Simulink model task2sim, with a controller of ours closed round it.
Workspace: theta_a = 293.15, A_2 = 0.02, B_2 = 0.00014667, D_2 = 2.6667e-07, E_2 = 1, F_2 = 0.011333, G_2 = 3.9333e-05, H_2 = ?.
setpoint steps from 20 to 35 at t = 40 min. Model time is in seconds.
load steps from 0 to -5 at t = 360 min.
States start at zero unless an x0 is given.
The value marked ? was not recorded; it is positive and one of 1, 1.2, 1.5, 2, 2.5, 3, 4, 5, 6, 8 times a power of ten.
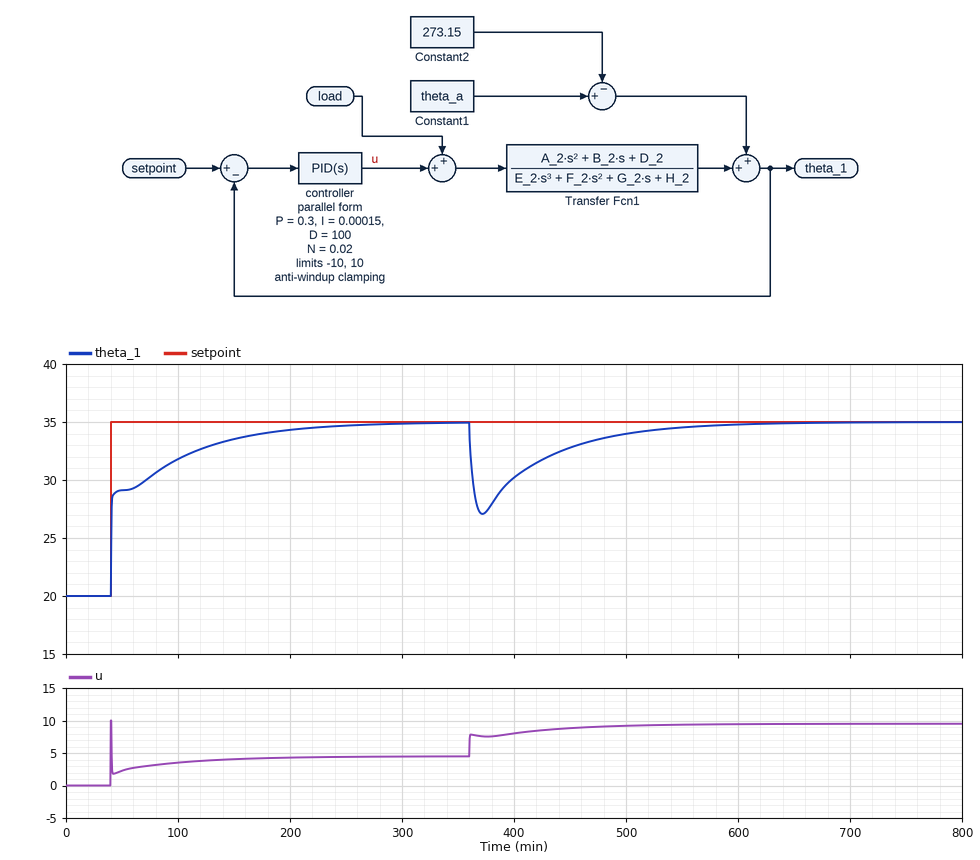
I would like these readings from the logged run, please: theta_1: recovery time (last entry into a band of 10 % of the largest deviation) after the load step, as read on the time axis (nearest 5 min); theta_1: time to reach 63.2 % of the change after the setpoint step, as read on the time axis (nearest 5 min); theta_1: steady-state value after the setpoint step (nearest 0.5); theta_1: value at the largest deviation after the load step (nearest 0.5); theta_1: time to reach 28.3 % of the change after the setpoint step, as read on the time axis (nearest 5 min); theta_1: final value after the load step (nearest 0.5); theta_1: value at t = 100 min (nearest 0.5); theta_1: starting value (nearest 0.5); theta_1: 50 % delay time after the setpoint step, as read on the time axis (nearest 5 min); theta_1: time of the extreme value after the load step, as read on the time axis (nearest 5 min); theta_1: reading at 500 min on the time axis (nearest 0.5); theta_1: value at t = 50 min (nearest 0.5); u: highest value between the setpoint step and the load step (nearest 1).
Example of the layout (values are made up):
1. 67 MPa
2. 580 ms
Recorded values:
1. 515 min
2. 65 min
3. 35.0
4. 27.0
5. 40 min
6. 35.0
7. 32.0
8. 20.0
9. 40 min
10. 370 min
11. 34.0
12. 29.0
13. 10
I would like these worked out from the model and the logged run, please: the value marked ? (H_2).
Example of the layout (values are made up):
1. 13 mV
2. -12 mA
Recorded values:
1. 8e-08
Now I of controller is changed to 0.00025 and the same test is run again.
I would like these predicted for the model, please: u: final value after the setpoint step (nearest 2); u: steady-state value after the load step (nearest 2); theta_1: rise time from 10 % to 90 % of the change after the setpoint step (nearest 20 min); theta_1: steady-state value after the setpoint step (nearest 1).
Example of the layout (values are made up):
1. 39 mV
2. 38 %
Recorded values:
1. 4
2. 10
3. 60 min
4. 35
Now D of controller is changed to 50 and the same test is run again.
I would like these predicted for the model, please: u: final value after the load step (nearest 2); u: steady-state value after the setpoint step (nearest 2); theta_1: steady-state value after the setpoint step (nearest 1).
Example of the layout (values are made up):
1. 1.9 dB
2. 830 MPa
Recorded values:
1. 10
2. 4
3. 35
